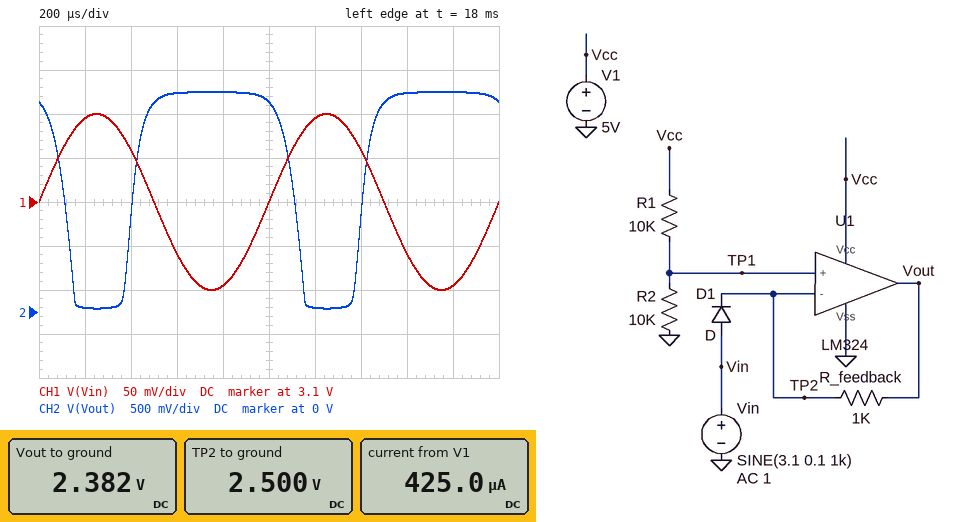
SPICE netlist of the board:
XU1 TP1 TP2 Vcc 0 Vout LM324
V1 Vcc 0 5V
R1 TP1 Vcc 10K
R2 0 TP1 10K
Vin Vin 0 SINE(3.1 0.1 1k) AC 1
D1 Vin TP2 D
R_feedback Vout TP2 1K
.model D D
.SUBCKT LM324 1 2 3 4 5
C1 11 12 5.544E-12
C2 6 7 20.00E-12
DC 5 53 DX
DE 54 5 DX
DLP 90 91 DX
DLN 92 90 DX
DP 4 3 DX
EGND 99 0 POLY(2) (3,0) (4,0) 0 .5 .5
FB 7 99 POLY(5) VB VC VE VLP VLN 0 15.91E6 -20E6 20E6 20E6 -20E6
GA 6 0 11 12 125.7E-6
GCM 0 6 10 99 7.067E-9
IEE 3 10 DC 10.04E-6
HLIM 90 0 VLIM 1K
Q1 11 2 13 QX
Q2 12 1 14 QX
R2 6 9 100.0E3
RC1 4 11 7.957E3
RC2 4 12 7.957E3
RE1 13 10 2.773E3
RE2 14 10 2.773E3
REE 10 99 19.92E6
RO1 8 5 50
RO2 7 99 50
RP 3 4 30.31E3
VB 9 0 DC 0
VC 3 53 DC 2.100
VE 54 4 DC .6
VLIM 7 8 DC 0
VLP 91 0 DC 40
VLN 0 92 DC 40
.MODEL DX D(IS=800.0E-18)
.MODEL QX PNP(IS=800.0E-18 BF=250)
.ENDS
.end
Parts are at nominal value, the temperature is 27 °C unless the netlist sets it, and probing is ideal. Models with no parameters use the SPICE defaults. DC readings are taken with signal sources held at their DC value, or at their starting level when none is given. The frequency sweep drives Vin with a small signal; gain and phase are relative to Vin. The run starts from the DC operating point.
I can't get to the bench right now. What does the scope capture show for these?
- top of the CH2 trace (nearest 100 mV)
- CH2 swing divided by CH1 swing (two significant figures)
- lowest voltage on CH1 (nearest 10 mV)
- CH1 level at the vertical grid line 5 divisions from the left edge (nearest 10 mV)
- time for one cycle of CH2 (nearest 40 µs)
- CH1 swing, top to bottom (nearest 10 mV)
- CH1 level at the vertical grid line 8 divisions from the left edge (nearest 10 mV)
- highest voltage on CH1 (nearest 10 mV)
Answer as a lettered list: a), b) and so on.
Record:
a) 2.5 V
b) 12
c) 3.00 V
d) 3.10 V
e) 1.00 ms
f) 200 mV
g) 3.04 V
h) 3.20 V
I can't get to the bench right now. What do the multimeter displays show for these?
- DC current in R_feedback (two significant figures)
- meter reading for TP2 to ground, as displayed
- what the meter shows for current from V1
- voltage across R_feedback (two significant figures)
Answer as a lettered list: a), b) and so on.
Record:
a) 120 µA
b) 2.500 V
c) 425.0 µA
d) 120 mV
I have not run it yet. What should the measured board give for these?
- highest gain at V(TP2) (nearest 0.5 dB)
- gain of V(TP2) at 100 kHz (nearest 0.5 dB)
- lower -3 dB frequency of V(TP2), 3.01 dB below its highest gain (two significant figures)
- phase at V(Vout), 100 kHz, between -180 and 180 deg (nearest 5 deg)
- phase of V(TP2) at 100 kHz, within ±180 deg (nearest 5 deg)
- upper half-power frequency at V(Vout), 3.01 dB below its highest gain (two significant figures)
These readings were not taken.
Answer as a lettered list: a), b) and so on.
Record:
a) -1.0 dB
b) -7.5 dB
c) 180 kHz
d) 150 deg
e) 60 deg
f) 190 kHz
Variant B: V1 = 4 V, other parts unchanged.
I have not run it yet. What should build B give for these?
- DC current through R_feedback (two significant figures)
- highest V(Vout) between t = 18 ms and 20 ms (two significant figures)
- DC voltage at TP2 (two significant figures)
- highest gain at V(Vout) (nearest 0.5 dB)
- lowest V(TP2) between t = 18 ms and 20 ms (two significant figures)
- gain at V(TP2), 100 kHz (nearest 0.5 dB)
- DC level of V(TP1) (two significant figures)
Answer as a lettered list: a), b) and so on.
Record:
a) 2.4 mA
b) 4.7 mV
c) 2.4 V
d) -58.0 dB
e) 2.3 V
f) 0 dB
g) 2.0 V
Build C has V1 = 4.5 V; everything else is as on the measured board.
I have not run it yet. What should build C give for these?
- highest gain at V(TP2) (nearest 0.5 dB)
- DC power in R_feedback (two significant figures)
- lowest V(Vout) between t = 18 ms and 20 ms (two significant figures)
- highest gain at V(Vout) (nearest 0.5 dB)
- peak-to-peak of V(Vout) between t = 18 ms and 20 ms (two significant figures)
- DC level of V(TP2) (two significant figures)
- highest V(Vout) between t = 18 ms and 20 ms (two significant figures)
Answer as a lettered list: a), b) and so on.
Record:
a) 0 dB
b) 5.8 mW
c) 4.7 mV
d) -42.5 dB
e) 7.0 mV
f) 2.4 V
g) 12 mV
